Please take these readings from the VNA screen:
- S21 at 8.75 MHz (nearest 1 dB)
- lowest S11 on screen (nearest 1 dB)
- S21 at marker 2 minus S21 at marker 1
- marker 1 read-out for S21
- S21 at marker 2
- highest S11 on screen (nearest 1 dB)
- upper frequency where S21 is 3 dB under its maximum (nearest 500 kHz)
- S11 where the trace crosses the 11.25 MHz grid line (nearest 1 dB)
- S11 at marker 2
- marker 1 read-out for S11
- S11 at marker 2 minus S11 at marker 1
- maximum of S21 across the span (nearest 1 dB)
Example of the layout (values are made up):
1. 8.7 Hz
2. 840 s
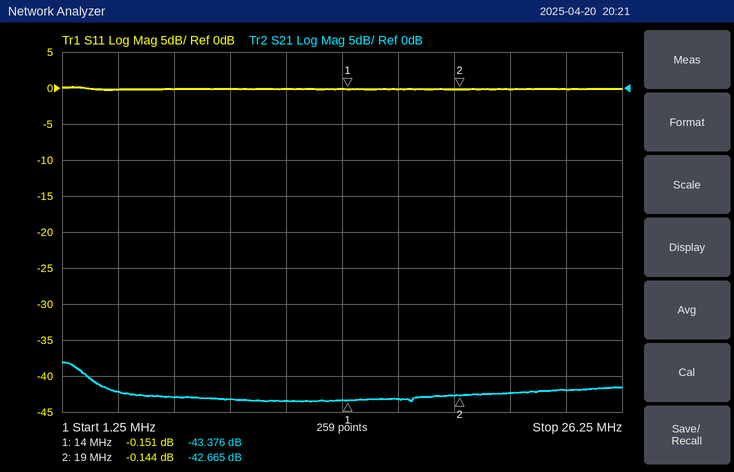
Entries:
1. -43 dB
2. 0 dB
3. 0.711 dB
4. -43.376 dB
5. -42.665 dB
6. 0 dB
7. 3.0 MHz
8. 0 dB
9. -0.144 dB
10. -0.151 dB
11. 0.007 dB
12. -38 dB
